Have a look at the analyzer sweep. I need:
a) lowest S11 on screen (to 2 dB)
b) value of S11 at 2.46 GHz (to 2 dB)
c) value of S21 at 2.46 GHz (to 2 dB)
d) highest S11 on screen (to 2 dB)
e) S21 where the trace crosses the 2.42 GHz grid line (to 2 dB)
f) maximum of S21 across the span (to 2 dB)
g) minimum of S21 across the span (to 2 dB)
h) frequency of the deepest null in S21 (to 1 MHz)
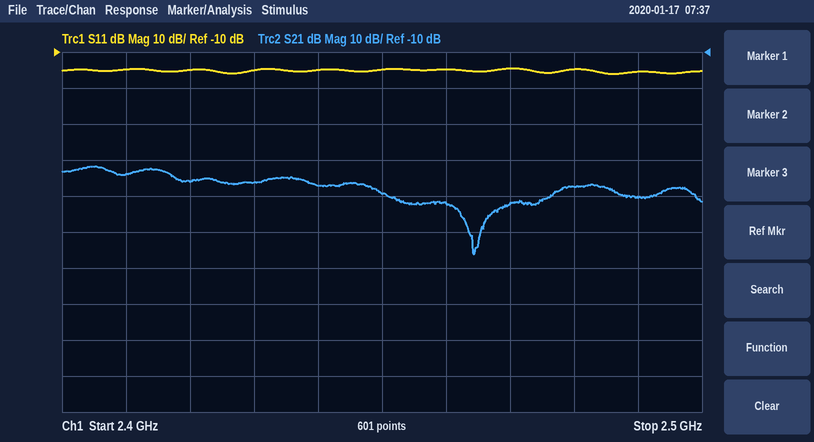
-16 dB
-14 dB
-52 dB
-14 dB
-46 dB
-42 dB
-66 dB
2.464 GHz
